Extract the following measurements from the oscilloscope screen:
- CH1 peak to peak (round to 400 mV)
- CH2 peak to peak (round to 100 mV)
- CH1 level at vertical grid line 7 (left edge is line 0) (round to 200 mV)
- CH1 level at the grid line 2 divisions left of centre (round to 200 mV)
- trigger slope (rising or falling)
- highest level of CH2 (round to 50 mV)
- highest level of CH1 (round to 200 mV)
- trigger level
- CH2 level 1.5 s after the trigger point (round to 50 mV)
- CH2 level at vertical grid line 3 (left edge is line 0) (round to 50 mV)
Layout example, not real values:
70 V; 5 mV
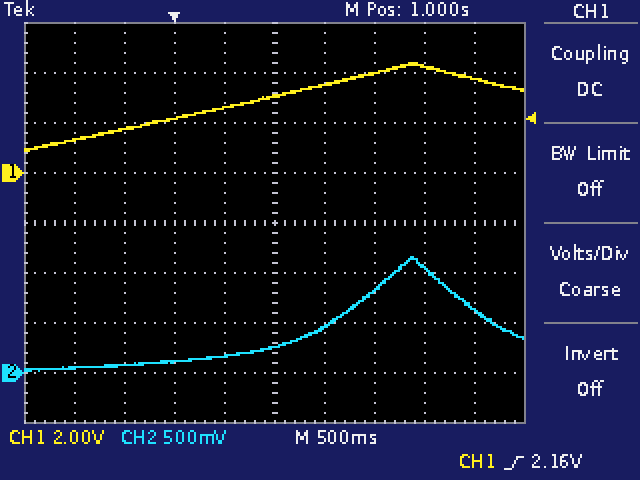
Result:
3.6 V; 1.10 V; 4.0 V; 2.2 V; rising; 1.15 V; 4.4 V; 2.16 V; 450 mV; 100 mV
